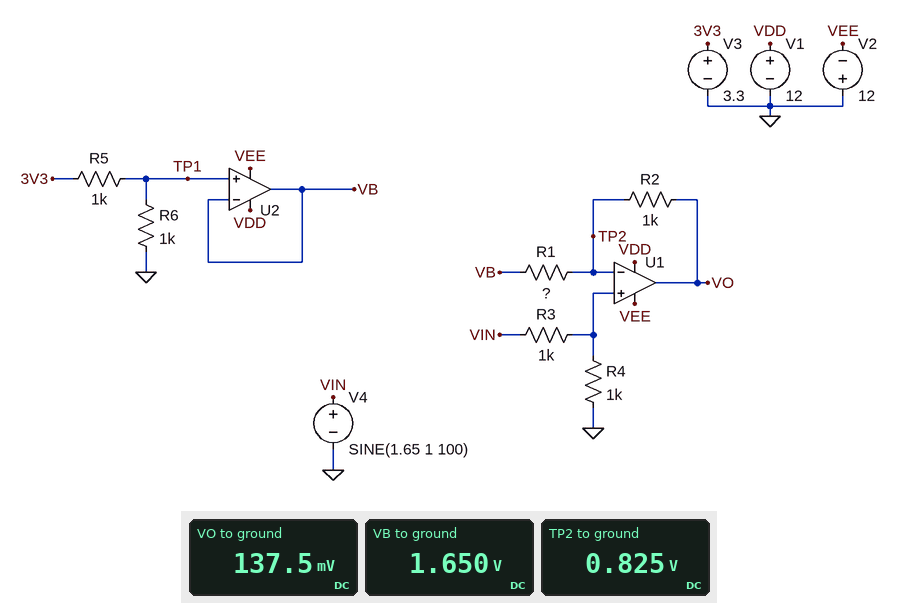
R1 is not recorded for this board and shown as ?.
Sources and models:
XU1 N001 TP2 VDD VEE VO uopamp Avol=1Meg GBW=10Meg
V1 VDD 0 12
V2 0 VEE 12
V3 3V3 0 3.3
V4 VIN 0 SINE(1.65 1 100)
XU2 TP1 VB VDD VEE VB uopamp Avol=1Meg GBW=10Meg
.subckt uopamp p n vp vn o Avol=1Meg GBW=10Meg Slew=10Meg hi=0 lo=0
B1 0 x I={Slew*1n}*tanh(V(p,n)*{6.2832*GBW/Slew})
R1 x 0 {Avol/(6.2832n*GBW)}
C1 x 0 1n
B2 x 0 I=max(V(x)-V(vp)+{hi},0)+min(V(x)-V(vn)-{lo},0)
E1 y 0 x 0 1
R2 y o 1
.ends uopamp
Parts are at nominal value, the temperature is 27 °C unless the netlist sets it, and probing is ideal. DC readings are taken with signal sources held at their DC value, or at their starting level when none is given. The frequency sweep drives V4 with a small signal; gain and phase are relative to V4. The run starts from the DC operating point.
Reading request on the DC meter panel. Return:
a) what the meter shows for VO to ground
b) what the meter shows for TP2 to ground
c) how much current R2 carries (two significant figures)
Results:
137.5 mV
0.825 V
690 µA
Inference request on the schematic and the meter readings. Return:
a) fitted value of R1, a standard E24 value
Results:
1.2 kΩ
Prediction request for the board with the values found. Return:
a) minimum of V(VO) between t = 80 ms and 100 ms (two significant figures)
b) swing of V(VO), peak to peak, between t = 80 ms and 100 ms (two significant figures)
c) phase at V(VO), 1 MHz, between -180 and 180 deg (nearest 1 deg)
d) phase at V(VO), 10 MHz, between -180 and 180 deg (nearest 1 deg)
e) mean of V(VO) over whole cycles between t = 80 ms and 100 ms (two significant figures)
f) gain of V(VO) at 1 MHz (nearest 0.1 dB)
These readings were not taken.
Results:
-780 mV
1.8 V
-10 deg
-61 deg
140 mV
-0.9 dB
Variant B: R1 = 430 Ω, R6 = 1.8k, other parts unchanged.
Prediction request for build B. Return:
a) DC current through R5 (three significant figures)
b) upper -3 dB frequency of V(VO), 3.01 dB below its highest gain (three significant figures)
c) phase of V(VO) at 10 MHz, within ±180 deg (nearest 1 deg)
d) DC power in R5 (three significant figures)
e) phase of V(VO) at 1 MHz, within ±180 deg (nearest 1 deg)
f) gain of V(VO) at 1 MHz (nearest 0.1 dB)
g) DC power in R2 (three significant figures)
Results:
1.18 mA
3.00 MHz
-73 deg
1.39 mW
-18 deg
4.0 dB
9.09 mW
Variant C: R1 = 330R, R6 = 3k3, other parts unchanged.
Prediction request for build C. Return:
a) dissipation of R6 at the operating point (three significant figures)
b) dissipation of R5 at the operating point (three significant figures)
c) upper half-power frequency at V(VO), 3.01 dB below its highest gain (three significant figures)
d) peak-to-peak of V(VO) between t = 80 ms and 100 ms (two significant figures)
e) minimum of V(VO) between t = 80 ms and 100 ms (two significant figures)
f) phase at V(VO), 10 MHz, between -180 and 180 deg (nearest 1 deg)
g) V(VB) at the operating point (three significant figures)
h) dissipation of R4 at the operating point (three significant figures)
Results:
1.94 mW
589 µW
2.48 MHz
4.0 V
-6.4 V
-76 deg
2.53 V
681 µW
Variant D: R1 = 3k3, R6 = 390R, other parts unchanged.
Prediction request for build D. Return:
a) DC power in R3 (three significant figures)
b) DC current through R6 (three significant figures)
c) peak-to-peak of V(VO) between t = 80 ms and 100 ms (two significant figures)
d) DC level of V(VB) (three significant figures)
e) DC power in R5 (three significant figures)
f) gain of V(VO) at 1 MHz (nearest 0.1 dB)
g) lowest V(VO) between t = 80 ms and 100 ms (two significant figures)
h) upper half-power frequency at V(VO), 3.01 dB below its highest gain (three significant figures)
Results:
681 µW
2.37 mA
1.3 V
926 mV
5.64 mW
-3.8 dB
140 mV
7.67 MHz
